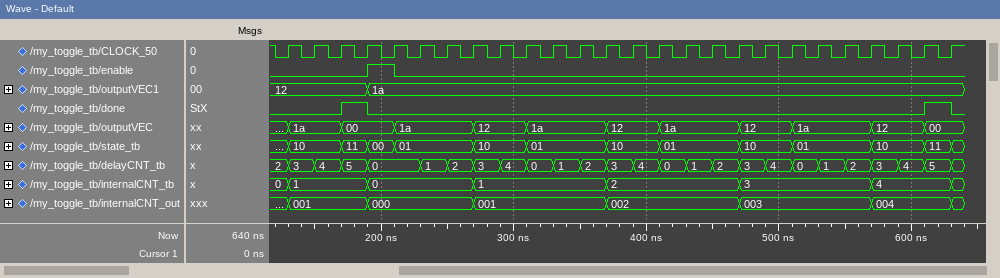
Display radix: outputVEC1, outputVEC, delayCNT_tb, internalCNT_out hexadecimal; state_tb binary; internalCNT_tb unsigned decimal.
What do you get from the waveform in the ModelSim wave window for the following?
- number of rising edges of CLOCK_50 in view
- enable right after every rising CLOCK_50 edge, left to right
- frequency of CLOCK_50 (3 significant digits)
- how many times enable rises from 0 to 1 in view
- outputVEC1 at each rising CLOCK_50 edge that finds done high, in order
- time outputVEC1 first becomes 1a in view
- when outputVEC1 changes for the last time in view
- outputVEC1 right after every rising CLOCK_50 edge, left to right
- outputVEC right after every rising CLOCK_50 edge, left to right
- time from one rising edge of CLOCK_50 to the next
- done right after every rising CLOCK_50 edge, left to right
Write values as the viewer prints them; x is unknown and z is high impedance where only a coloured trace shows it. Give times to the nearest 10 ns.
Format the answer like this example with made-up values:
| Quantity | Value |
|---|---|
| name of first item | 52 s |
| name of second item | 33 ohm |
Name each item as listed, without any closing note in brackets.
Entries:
| Quantity | Value |
|---|---|
| number of rising edges of CLOCK_50 in view | 26 |
| enable right after every rising CLOCK_50 edge, left to right | 0 0 0 1 0 0 0 0 0 0 0 0 0 0 0 0 0 0 0 0 0 0 0 0 0 0 |
| frequency of CLOCK_50 | 50.0 MHz |
| how many times enable rises from 0 to 1 in view | 1 |
| outputVEC1 at each rising CLOCK_50 edge that finds done high, in order | 12, 1a |
| time outputVEC1 first becomes 1a in view | 190 ns |
| when outputVEC1 changes for the last time in view | 190 ns |
| outputVEC1 right after every rising CLOCK_50 edge, left to right | 12, 12, 12, 1a, 1a, 1a, 1a, 1a, 1a, 1a, 1a, 1a, 1a, 1a, 1a, 1a, 1a, 1a, 1a, 1a, 1a, 1a, 1a, 1a, 1a, 1a |
| outputVEC right after every rising CLOCK_50 edge, left to right | 1a, 1a, 00, 00, 1a, 1a, 1a, 12, 12, 1a, 1a, 1a, 12, 12, 1a, 1a, 1a, 12, 12, 1a, 1a, 1a, 12, 12, 00, 00 |
| time from one rising edge of CLOCK_50 to the next | 20 ns |
| done right after every rising CLOCK_50 edge, left to right | 0 0 1 0 0 0 0 0 0 0 0 0 0 0 0 0 0 0 0 0 0 0 0 0 1 0 |
